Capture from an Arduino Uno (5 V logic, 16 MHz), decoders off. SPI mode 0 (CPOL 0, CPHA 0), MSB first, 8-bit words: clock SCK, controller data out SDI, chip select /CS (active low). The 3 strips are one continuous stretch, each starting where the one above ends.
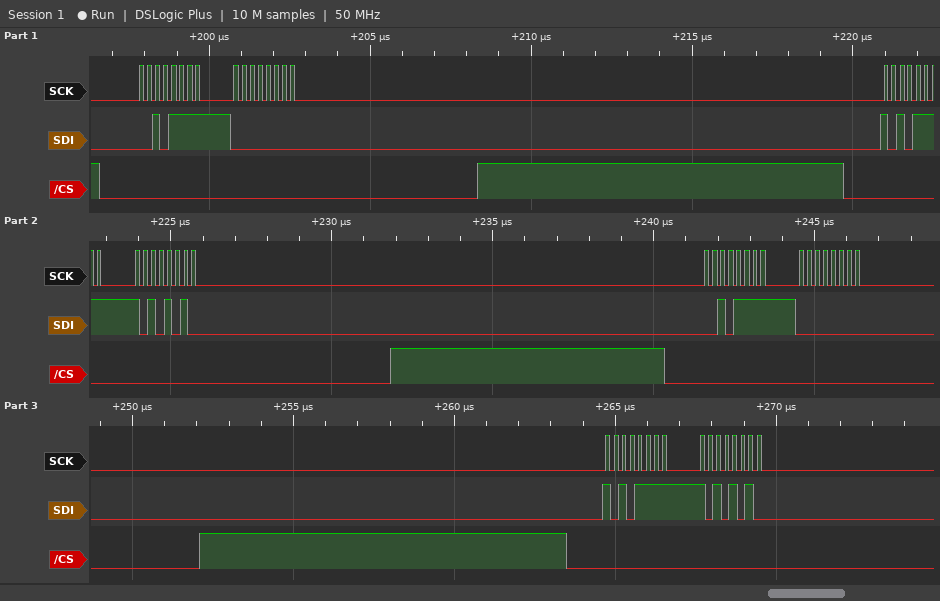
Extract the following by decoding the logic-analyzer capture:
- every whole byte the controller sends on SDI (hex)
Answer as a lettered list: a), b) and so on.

a) 2F 00 AF AA 2F 00 AF AA
